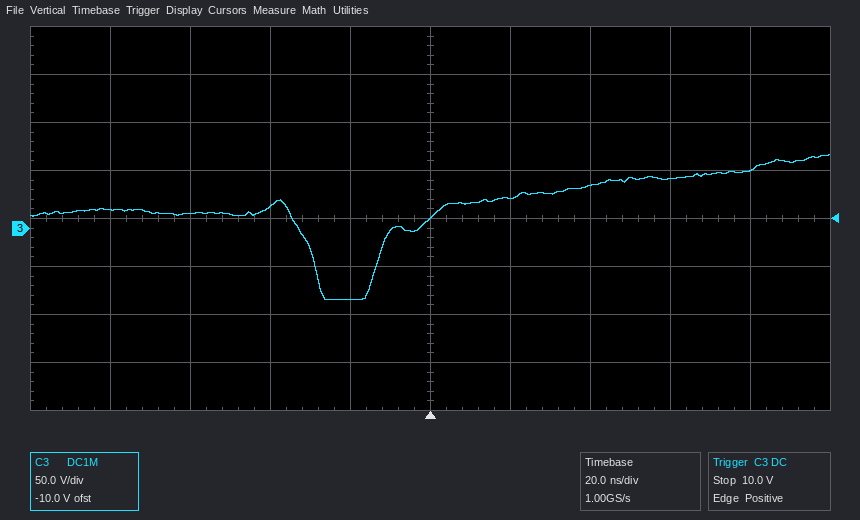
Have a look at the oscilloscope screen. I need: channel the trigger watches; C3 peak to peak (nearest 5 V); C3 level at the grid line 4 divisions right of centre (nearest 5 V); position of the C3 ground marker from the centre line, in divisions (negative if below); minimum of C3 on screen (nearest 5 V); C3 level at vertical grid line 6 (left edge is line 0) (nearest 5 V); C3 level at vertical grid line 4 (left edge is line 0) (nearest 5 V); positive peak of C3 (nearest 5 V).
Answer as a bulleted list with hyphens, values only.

- C3
- 150 V
- 60 V
- -0.2 div
- -75 V
- 30 V
- -75 V
- 75 V
